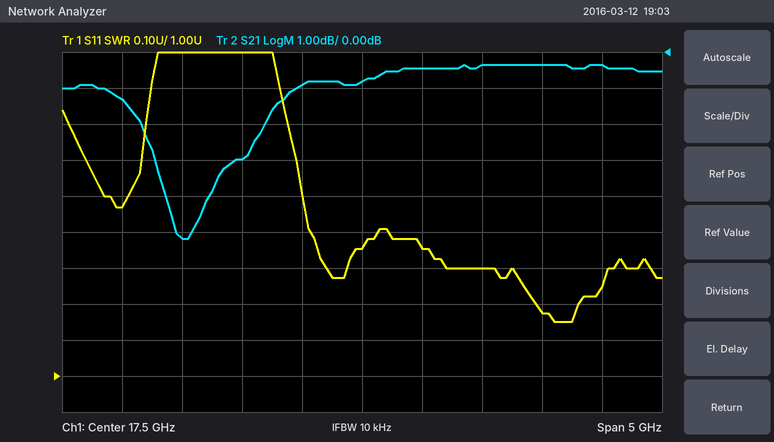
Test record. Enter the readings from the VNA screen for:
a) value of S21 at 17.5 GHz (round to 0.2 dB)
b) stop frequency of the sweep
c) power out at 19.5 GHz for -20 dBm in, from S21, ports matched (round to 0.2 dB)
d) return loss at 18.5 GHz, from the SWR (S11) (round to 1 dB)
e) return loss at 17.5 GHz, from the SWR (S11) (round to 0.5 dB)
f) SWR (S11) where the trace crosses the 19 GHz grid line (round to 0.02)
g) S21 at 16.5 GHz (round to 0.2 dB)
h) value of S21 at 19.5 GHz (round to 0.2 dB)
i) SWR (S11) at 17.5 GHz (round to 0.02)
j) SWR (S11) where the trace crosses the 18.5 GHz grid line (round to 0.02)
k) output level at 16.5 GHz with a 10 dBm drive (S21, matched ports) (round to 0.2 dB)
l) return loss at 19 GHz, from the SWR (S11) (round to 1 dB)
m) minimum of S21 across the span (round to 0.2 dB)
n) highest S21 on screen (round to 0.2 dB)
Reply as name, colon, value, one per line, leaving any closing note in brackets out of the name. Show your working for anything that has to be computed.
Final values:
value of S21 at 17.5 GHz: -0.8 dB
stop frequency of the sweep: 20 GHz
power out at 19.5 GHz for -20 dBm in, from S21, ports matched: -20 dBm + (-0.4 dB) = -20.4 dBm
return loss at 18.5 GHz, from the SWR (S11): −20 log10((1.3 − 1)/(1.3 + 1)) ≈ 18 dB
return loss at 17.5 GHz, from the SWR (S11): −20 log10((1.36 − 1)/(1.36 + 1)) ≈ 16.3 dB, so 16.5 dB to the nearest 0.5 dB
SWR (S11) where the trace crosses the 19 GHz grid line: 1.18
S21 at 16.5 GHz: -3.0 dB
value of S21 at 19.5 GHz: -0.4 dB
SWR (S11) at 17.5 GHz: 1.36
SWR (S11) where the trace crosses the 18.5 GHz grid line: 1.30
output level at 16.5 GHz with a 10 dBm drive (S21, matched ports): 10 dBm + (-3.0 dB) = 7.0 dBm
return loss at 19 GHz, from the SWR (S11): −20 log10((1.18 − 1)/(1.18 + 1)) ≈ 22 dB
minimum of S21 across the span: -5.2 dB
highest S21 on screen: -0.4 dB
